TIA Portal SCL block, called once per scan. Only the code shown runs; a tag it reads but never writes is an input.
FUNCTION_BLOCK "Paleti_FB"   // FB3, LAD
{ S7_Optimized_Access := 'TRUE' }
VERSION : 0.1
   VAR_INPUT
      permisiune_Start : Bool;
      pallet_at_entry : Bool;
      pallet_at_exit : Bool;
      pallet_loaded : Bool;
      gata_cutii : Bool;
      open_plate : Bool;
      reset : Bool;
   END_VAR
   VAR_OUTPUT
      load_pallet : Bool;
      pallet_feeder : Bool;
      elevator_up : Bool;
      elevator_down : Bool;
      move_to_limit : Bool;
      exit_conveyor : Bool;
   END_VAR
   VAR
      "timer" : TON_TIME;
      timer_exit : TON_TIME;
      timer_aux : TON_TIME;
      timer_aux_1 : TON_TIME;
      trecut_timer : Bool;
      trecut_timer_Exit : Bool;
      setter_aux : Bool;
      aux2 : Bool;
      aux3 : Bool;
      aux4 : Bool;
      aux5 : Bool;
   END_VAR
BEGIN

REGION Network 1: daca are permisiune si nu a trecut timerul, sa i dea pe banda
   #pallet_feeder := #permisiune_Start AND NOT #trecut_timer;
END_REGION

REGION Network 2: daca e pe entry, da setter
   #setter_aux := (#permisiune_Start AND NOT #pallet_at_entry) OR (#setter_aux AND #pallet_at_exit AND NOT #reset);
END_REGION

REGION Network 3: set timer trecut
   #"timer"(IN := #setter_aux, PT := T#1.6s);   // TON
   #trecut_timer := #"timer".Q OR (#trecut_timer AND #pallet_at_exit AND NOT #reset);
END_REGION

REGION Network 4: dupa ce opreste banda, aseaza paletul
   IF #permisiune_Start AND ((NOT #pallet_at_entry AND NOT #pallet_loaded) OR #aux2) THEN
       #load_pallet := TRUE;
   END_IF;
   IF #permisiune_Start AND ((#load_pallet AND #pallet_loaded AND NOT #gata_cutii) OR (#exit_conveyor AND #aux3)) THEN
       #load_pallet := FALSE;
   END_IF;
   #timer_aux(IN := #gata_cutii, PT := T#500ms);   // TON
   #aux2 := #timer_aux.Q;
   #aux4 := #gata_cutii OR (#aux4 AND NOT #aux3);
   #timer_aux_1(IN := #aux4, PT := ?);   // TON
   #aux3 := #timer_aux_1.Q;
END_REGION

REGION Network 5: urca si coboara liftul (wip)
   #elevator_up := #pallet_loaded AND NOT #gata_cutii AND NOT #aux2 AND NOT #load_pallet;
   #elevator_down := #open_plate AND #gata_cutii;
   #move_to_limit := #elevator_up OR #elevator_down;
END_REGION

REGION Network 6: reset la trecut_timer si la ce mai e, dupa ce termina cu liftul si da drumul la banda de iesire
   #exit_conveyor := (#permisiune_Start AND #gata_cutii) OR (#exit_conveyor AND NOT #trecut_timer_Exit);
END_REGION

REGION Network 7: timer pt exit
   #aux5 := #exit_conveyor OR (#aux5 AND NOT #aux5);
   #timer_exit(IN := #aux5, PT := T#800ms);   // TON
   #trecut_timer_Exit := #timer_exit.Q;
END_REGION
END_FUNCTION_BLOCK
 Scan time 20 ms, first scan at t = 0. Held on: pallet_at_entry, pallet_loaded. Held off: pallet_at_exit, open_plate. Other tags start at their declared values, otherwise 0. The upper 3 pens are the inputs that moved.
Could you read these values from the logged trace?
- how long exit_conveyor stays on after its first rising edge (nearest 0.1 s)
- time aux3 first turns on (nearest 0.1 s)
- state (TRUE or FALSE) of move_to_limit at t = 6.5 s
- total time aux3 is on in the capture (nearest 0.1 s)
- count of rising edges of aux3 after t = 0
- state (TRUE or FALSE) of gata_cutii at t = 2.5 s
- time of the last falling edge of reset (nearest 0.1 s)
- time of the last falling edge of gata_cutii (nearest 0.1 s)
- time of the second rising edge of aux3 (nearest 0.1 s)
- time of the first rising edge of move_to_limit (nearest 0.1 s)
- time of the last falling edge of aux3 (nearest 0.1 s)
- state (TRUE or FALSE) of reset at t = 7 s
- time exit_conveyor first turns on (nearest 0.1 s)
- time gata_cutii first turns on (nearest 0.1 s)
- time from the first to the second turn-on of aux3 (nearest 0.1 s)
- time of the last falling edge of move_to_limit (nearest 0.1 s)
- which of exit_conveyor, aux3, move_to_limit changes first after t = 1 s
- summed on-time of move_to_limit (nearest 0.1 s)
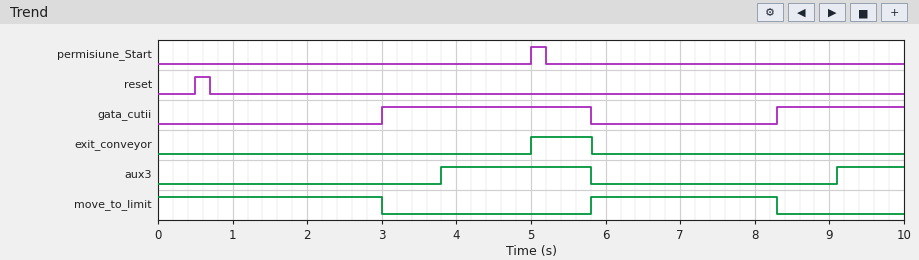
0.8 s
3.8 s
TRUE
2.9 s
2
FALSE
0.7 s
5.8 s
9.1 s
5.8 s
5.8 s
FALSE
5.0 s
3.0 s
5.3 s
8.3 s
move_to_limit
5.5 s
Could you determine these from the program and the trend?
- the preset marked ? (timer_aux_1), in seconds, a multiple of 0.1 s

0.8 s
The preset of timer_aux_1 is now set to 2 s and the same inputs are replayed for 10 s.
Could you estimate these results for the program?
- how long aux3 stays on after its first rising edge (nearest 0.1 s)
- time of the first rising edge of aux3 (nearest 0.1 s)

0.8 s
5.0 s
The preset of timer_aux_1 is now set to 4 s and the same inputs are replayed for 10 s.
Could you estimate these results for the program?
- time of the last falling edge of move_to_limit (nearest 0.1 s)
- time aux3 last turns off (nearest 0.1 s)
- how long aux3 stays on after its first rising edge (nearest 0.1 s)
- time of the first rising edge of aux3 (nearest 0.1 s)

3.0 s
7.0 s
0.0 s
7.0 s
